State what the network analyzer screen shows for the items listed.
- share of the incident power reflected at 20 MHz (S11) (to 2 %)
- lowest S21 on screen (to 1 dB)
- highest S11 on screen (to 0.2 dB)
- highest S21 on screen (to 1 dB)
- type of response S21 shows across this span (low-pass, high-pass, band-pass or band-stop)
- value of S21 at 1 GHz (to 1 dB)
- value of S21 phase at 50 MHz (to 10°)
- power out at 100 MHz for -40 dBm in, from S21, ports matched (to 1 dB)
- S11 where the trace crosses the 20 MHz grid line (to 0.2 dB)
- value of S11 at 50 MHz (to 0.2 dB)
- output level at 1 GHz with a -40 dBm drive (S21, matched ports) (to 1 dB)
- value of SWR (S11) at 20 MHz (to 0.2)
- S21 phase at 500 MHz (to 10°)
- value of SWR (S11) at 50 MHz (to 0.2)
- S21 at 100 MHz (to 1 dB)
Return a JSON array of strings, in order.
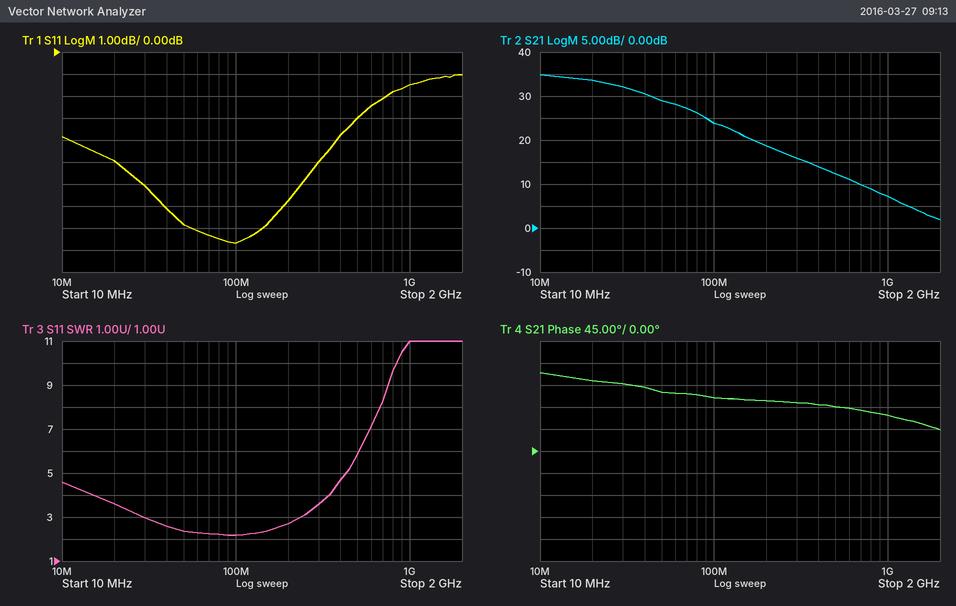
["32 %", "2 dB", "-1.0 dB", "35 dB", "low-pass", "7 dB", "120°", "-16 dBm", "-5.0 dB", "-7.8 dB", "-33 dBm", "3.6", "90°", "2.4", "24 dB"]
